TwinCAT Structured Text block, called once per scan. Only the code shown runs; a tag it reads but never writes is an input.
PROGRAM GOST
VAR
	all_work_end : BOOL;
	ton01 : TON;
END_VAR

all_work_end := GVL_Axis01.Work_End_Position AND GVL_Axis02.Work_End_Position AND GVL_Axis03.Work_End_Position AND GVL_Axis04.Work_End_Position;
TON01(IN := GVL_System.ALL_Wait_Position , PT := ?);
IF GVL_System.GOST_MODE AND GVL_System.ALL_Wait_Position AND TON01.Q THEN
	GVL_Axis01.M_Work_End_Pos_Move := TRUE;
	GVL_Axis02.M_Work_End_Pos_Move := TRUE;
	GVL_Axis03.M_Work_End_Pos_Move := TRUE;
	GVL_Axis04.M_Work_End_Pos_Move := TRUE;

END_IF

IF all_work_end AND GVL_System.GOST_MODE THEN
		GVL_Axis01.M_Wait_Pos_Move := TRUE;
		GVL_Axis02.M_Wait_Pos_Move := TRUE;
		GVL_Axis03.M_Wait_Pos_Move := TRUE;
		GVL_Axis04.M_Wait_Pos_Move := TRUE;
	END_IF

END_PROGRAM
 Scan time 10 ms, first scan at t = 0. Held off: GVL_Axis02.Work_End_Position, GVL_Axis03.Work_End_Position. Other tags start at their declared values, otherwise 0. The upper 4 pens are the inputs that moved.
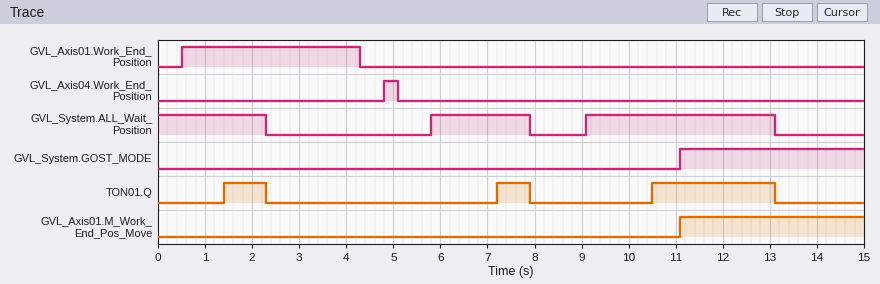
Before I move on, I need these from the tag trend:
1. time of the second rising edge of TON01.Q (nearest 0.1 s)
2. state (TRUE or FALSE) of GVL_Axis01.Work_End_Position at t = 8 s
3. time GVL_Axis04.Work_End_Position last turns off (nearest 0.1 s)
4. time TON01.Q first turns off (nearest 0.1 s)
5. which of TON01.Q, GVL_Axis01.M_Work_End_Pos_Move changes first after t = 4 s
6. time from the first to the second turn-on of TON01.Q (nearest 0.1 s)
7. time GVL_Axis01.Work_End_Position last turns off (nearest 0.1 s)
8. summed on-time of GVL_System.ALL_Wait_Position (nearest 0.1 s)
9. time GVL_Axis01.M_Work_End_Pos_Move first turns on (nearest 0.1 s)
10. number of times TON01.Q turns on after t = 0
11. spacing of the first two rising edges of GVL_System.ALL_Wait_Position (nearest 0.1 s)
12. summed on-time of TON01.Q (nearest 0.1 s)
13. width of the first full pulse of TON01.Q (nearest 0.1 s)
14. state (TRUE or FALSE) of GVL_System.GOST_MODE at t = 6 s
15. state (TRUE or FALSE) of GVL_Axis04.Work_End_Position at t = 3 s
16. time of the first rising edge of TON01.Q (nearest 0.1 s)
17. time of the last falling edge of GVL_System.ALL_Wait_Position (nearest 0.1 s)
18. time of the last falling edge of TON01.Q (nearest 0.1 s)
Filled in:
7.2 s
FALSE
5.1 s
2.3 s
TON01.Q
5.8 s
4.3 s
8.4 s
11.1 s
3
3.3 s
4.2 s
0.9 s
FALSE
FALSE
1.4 s
13.1 s
13.1 s
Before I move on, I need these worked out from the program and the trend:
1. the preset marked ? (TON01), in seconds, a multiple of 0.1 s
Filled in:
1.4 s
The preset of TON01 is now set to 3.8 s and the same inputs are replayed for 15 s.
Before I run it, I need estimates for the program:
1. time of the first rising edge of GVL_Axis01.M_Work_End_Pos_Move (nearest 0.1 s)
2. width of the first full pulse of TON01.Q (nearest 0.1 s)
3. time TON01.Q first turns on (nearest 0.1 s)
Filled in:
12.9 s
0.2 s
12.9 s
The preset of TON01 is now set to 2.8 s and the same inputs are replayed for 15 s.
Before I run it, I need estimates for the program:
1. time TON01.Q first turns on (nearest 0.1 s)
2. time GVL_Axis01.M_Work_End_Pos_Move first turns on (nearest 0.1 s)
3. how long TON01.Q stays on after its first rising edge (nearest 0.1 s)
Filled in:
11.9 s
11.9 s
1.2 s
